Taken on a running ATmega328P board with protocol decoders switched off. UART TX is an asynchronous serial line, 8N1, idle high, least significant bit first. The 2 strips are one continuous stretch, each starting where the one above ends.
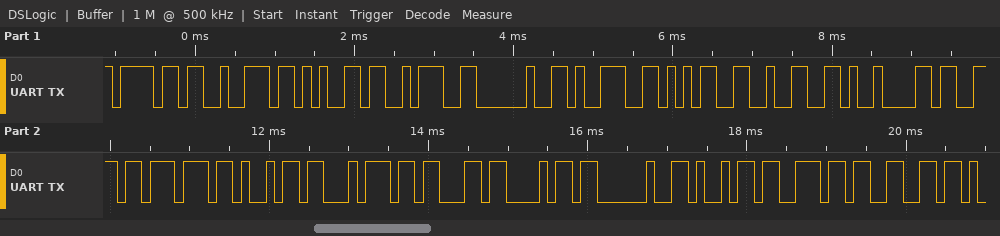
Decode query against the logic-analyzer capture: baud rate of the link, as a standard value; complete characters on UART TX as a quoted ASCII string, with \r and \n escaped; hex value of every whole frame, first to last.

9600 baud
"ore: 952\tswitch inf"
6F 72 65 3A 20 39 35 32 09 73 77 69 74 63 68 20 69 6E 66
